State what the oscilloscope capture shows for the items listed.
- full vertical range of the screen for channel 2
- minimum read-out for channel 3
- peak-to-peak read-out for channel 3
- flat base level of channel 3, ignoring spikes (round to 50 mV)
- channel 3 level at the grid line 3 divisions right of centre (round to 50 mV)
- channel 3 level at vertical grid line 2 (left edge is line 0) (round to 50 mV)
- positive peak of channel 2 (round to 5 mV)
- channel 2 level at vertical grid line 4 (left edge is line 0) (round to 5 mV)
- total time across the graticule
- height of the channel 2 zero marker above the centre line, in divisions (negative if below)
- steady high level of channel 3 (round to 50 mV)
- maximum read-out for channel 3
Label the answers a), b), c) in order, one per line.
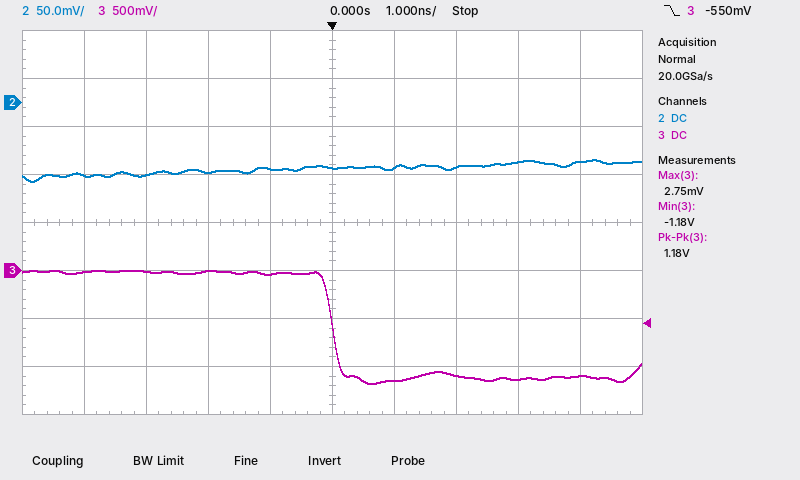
a) 400 mV
b) -1.18 V
c) 1.18 V
d) -1.10 V
e) -1.15 V
f) 0 mV
g) -60 mV
h) -70 mV
i) 10 ns
j) +2.5 div
k) 0 mV
l) 2.75 mV
